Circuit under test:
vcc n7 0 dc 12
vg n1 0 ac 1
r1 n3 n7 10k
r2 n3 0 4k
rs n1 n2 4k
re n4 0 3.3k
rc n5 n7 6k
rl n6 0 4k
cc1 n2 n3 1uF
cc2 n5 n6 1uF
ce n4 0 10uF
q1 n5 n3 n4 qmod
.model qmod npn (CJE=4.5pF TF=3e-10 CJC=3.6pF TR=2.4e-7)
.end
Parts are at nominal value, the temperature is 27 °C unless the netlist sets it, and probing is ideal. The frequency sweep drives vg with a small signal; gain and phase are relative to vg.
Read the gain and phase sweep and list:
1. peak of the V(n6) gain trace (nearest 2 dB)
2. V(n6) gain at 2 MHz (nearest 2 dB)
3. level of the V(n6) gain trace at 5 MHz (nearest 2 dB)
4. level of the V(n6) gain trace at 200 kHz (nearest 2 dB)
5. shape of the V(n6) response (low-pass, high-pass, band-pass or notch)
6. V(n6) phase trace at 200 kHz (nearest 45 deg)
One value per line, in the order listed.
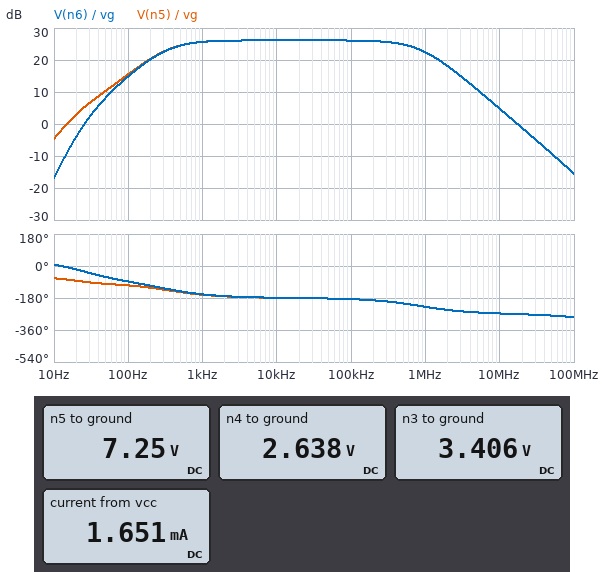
26 dB
18 dB
10 dB
26 dB
band-pass
-180 deg
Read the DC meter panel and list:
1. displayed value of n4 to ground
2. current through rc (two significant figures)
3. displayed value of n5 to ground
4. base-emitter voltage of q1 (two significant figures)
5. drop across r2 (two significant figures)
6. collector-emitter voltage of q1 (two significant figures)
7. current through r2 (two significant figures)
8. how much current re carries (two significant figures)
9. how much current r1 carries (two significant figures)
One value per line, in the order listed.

2.638 V
790 µA
7.25 V
770 mV
3.4 V
4.6 V
850 µA
800 µA
860 µA
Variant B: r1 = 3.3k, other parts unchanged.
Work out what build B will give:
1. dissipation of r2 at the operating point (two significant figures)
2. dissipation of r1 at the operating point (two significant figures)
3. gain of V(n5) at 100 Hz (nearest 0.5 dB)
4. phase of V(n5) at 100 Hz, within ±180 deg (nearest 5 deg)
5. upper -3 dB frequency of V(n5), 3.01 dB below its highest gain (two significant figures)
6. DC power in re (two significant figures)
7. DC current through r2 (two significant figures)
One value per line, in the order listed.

8.6 mW
11 mW
-29.0 dB
-70 deg
74 Hz
7.8 mW
1.5 mA
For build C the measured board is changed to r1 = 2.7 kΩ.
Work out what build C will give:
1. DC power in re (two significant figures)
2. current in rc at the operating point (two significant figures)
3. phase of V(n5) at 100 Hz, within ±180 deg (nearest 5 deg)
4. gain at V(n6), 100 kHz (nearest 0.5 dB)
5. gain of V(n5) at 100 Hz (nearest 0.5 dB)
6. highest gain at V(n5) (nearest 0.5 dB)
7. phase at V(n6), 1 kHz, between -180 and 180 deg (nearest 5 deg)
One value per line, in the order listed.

9.0 mW
1.1 mA
-65 deg
-45.0 dB
-29.5 dB
-24.5 dB
-140 deg
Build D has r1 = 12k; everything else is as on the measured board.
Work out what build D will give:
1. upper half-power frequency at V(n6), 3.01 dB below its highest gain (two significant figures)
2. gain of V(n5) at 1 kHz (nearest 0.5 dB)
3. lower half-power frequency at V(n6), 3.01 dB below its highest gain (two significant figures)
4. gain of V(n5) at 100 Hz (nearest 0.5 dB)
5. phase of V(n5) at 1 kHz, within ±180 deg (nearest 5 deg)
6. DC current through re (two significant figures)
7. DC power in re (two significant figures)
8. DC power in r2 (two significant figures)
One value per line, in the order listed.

1.0 MHz
25.0 dB
300 Hz
15.5 dB
-165 deg
670 µA
1.5 mW
2.2 mW
